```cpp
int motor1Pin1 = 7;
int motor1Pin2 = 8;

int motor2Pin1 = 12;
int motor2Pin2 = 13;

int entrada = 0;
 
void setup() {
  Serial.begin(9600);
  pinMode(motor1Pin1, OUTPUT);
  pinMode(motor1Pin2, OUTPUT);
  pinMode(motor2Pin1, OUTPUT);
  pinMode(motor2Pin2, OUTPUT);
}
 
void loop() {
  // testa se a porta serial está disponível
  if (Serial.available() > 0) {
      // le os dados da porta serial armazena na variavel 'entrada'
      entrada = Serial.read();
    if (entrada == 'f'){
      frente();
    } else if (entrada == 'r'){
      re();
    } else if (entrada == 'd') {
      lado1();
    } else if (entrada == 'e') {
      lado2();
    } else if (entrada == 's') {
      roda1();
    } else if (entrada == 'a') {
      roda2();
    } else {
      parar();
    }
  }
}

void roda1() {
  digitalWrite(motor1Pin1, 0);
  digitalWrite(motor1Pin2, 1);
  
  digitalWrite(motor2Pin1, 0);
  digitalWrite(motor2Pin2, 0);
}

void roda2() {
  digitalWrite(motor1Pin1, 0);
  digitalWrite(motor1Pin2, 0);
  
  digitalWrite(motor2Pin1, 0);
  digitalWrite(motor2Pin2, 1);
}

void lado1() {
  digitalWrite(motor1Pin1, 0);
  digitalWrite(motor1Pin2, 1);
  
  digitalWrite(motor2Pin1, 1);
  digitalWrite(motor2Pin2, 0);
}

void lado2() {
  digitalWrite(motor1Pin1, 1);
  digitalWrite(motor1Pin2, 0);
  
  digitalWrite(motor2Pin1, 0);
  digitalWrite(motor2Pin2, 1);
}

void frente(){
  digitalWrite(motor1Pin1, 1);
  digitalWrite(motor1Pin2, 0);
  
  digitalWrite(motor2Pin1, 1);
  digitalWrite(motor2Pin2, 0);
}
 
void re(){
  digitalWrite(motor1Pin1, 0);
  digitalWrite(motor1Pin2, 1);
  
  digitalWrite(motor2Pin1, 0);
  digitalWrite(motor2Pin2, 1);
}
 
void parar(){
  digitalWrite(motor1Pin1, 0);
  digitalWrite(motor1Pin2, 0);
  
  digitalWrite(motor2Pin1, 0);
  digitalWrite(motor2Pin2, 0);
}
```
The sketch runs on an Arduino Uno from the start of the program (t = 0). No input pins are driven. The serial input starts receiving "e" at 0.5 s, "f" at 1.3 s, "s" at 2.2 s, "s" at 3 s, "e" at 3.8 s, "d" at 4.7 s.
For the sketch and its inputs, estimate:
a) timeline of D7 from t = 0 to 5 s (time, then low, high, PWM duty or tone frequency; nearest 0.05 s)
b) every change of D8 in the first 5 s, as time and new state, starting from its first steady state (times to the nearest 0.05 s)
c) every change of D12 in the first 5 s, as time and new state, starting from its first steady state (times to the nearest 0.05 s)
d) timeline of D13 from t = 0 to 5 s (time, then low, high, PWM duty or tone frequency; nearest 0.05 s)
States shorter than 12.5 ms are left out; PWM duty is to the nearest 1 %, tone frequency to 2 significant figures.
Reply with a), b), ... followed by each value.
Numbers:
a) 0 s low; 0.5 s high; 2.2 s low; 3.8 s high; 4.7 s low
b) 0 s low; 2.2 s high; 3.8 s low; 4.7 s high
c) 0 s low; 1.3 s high; 2.2 s low; 4.7 s high
d) 0 s low; 0.5 s high; 1.3 s low; 3.8 s high; 4.7 s low
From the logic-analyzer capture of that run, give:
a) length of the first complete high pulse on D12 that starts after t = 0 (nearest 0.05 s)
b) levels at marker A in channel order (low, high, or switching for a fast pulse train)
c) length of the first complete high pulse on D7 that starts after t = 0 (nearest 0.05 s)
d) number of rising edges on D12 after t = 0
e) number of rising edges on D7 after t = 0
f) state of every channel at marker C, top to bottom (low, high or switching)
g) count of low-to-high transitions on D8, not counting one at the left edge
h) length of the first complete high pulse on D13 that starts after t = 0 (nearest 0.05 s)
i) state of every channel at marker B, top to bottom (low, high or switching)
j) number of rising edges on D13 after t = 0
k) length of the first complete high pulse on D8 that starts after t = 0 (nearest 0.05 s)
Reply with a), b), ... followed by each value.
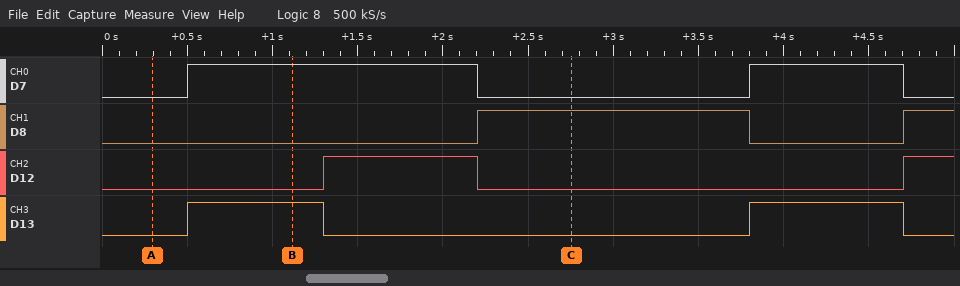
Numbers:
a) 0.90 s
b) D7 low, D8 low, D12 low, D13 low
c) 1.70 s
d) 2
e) 2
f) D7 low, D8 high, D12 low, D13 low
g) 2
h) 0.80 s
i) D7 high, D8 low, D12 low, D13 high
j) 2
k) 1.60 s
